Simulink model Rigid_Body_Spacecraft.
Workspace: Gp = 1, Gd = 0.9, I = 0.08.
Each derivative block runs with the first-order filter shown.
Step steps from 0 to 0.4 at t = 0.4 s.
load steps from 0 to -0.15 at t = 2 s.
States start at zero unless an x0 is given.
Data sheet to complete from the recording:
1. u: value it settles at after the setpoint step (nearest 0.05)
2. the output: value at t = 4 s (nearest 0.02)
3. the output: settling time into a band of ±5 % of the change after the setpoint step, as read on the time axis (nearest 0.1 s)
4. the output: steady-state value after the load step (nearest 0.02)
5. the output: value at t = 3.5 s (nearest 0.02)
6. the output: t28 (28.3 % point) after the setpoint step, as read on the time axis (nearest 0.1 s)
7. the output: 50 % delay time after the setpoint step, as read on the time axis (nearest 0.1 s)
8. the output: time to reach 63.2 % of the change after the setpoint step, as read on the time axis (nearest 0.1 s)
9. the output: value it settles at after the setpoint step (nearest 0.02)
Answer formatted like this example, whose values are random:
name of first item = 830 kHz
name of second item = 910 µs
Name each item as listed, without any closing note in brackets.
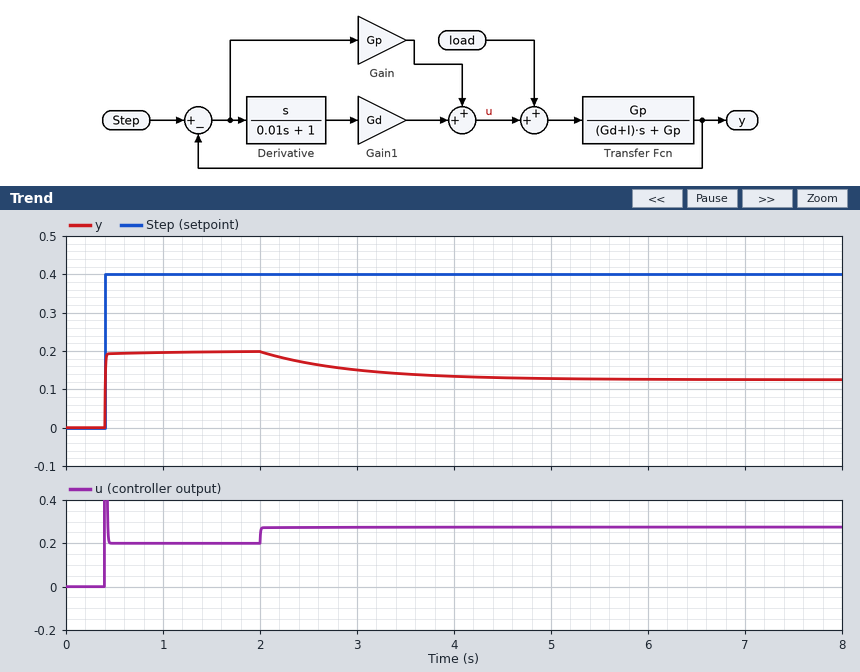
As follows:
u: value it settles at after the setpoint step = 0.20
the output: value at t = 4 s = 0.14
the output: settling time into a band of ±5 % of the change after the setpoint step, as read on the time axis = 0.4 s
the output: steady-state value after the load step = 0.12
the output: value at t = 3.5 s = 0.14
the output: t28 (28.3 % point) after the setpoint step, as read on the time axis = 0.4 s
the output: 50 % delay time after the setpoint step, as read on the time axis = 0.4 s
the output: time to reach 63.2 % of the change after the setpoint step, as read on the time axis = 0.4 s
the output: value it settles at after the setpoint step = 0.20
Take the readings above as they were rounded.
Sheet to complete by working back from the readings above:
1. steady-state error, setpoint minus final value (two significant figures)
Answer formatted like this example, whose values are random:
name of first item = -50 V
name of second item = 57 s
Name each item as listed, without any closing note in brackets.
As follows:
steady-state error, setpoint minus final value = 0.20
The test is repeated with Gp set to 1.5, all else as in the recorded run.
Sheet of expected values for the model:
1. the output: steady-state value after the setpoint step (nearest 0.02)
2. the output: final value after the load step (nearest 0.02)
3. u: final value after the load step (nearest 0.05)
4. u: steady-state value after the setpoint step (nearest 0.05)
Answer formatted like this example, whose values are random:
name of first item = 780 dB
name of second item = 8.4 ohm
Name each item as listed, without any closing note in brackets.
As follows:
the output: steady-state value after the setpoint step = 0.24
the output: final value after the load step = 0.18
u: final value after the load step = 0.35
u: steady-state value after the setpoint step = 0.25
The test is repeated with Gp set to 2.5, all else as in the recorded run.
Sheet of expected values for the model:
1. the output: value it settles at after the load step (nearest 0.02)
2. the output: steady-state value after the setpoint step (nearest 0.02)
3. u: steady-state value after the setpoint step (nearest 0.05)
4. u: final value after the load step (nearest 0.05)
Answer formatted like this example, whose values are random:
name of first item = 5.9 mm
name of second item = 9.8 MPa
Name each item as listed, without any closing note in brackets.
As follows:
the output: value it settles at after the load step = 0.24
the output: steady-state value after the setpoint step = 0.28
u: steady-state value after the setpoint step = 0.30
u: final value after the load step = 0.40
